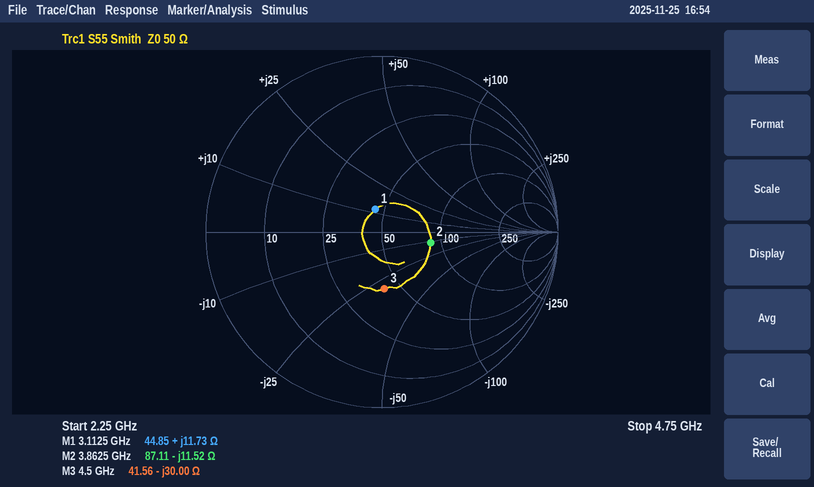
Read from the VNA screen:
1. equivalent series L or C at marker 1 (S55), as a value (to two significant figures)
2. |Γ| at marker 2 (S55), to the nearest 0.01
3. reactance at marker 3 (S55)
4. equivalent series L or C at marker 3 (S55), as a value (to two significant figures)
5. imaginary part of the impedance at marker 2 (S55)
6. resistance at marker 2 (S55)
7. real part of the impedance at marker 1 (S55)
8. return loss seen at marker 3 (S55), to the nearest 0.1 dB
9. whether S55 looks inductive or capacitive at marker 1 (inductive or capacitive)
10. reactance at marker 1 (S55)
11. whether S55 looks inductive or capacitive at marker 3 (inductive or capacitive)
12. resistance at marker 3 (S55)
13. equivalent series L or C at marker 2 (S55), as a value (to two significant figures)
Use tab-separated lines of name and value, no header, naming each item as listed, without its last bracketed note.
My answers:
equivalent series L or C at marker 1 (S55), as a value	600 pH
|Γ| at marker 2 (S55), to the nearest 0.01	0.28
reactance at marker 3	-30.00 Ω
equivalent series L or C at marker 3 (S55), as a value	1.2 pF
imaginary part of the impedance at marker 2	-11.52 Ω
resistance at marker 2	87.11 Ω
real part of the impedance at marker 1	44.85 Ω
return loss seen at marker 3 (S55), to the nearest 0.1 dB	9.8 dB
whether S55 looks inductive or capacitive at marker 1	inductive
reactance at marker 1	+11.73 Ω
whether S55 looks inductive or capacitive at marker 3	capacitive
resistance at marker 3	41.56 Ω
equivalent series L or C at marker 2 (S55), as a value	3.6 pF
